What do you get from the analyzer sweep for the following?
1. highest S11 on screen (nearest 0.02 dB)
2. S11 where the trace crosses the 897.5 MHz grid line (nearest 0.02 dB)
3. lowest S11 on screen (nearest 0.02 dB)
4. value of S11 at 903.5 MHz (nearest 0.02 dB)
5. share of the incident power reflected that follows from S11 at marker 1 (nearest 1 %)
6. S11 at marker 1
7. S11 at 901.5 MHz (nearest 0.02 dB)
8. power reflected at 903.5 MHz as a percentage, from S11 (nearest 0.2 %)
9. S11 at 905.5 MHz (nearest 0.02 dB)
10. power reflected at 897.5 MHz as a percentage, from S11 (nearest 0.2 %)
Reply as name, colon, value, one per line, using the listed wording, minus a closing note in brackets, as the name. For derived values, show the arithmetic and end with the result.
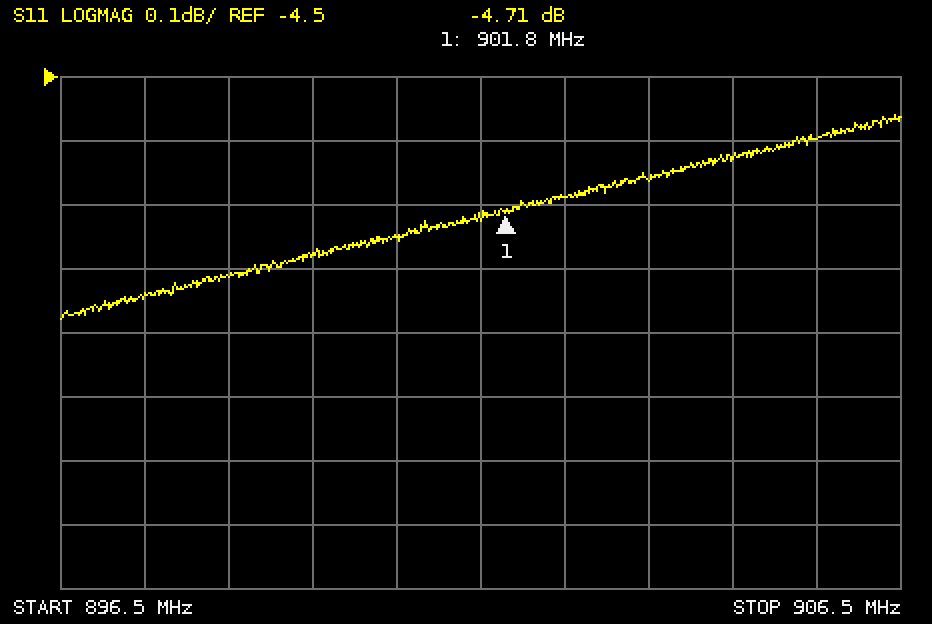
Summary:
highest S11 on screen: -4.56 dB
S11 where the trace crosses the 897.5 MHz grid line: -4.84 dB
lowest S11 on screen: -4.88 dB
value of S11 at 903.5 MHz: -4.66 dB
share of the incident power reflected that follows from S11 at marker 1: 10^(-4.71/10) ≈ 34 %
S11 at marker 1: -4.71 dB
S11 at 901.5 MHz: -4.72 dB
power reflected at 903.5 MHz as a percentage, from S11: 10^(-4.66/10) ≈ 34.2 %
S11 at 905.5 MHz: -4.60 dB
power reflected at 897.5 MHz as a percentage, from S11: 10^(-4.84/10) ≈ 32.8 %
